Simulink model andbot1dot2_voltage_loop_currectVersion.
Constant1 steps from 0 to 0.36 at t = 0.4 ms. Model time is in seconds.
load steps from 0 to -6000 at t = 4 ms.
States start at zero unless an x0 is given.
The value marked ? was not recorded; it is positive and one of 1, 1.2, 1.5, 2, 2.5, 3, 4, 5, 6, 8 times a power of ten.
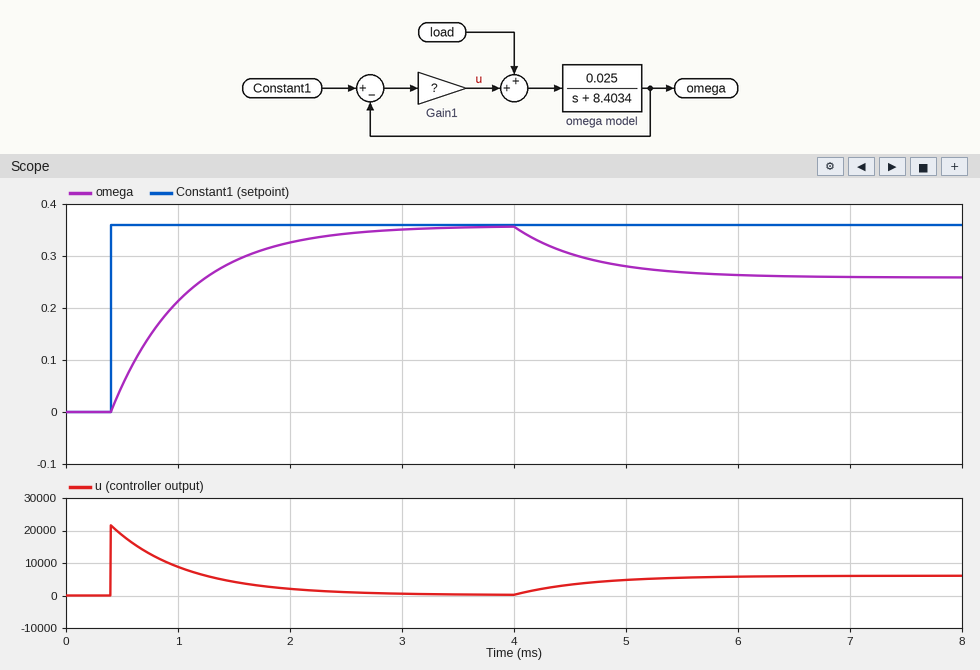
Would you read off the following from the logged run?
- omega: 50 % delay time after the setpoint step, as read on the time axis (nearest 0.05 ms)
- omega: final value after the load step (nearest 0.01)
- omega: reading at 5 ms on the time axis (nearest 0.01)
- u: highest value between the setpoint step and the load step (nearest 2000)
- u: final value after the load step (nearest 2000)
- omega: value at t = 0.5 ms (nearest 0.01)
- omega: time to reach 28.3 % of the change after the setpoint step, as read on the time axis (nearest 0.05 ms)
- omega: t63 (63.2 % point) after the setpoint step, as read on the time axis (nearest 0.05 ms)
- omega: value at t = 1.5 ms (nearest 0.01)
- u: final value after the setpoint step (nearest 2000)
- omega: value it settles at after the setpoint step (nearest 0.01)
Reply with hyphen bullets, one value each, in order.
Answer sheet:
- 0.85 ms
- 0.26
- 0.28
- 22000
- 6000
- 0.05
- 0.60 ms
- 1.05 ms
- 0.29
- 0
- 0.36
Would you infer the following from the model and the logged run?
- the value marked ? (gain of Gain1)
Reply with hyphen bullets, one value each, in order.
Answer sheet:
- 60000
